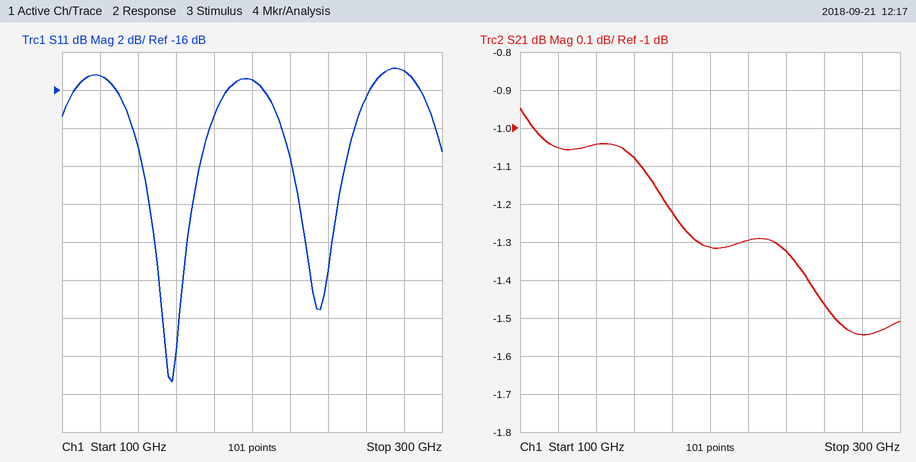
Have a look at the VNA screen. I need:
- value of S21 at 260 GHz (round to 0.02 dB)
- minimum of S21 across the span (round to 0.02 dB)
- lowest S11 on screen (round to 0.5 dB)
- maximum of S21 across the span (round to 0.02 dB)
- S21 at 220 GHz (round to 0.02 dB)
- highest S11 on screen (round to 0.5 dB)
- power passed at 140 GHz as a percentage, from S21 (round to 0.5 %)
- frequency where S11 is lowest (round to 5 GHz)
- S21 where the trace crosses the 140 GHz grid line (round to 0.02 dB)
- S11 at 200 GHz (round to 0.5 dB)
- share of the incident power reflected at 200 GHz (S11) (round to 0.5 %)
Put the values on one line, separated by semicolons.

-1.46 dB; -1.54 dB; -31.5 dB; -0.94 dB; -1.30 dB; -15.0 dB; 78.5 %; 160 GHz; -1.04 dB; -15.5 dB; 3.0 %
